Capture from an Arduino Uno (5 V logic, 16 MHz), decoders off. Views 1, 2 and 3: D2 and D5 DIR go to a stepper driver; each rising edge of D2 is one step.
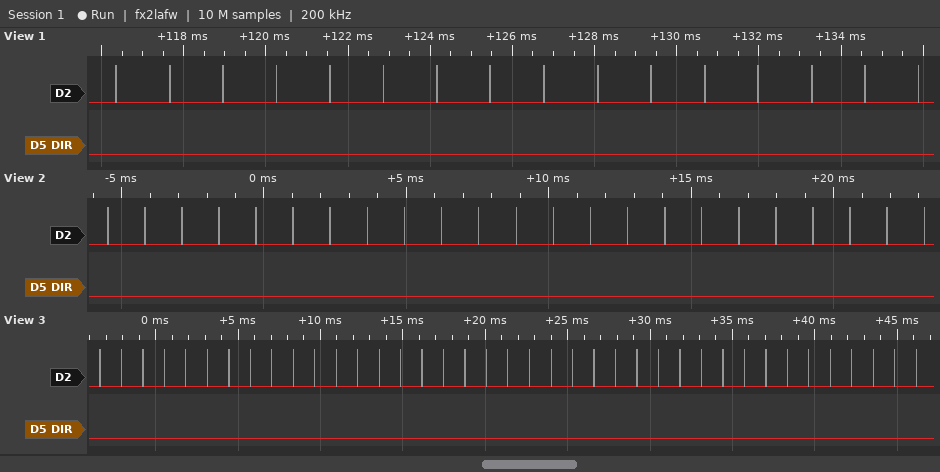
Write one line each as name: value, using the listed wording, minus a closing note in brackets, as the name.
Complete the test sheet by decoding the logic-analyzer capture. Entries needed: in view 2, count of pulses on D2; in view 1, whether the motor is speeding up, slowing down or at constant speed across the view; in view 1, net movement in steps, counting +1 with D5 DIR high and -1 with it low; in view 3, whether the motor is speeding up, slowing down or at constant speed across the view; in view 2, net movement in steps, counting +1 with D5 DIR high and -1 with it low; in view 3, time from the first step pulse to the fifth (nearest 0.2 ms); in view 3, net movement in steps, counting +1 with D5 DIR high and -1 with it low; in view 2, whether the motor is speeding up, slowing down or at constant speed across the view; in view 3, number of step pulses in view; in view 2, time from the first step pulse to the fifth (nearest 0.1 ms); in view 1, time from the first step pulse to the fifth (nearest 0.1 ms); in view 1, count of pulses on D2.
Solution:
in view 2, count of pulses on D2: 23
in view 1, whether the motor is speeding up, slowing down or at constant speed across the view: constant speed
in view 1, net movement in steps, counting +1 with D5 DIR high and -1 with it low: -16
in view 3, whether the motor is speeding up, slowing down or at constant speed across the view: constant speed
in view 2, net movement in steps, counting +1 with D5 DIR high and -1 with it low: -23
in view 3, time from the first step pulse to the fifth: 5.2 ms
in view 3, net movement in steps, counting +1 with D5 DIR high and -1 with it low: -39
in view 2, whether the motor is speeding up, slowing down or at constant speed across the view: constant speed
in view 3, number of step pulses in view: 39
in view 2, time from the first step pulse to the fifth: 5.2 ms
in view 1, time from the first step pulse to the fifth: 5.2 ms
in view 1, count of pulses on D2: 16
